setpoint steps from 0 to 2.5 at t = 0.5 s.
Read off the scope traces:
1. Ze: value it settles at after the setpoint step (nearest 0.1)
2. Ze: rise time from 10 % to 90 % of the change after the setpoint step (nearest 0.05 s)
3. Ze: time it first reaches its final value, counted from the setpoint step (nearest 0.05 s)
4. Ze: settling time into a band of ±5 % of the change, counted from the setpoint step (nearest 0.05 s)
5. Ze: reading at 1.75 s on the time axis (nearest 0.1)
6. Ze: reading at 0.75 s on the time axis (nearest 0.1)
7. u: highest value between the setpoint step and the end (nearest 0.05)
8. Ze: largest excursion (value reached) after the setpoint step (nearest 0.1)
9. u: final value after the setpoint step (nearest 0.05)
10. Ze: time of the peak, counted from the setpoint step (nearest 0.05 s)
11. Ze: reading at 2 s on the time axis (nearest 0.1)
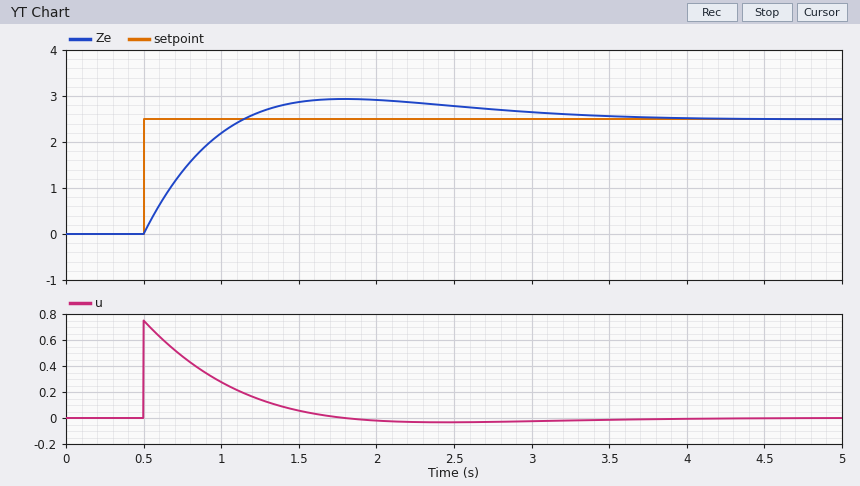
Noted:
2.5
0.50 s
0.65 s
2.60 s
2.9
1.4
0.75
2.9
0.00
1.30 s
2.9
